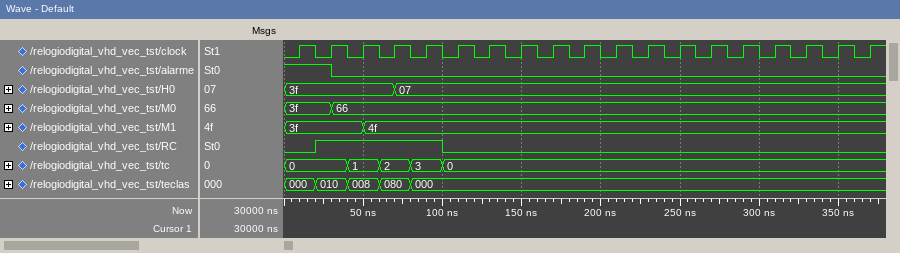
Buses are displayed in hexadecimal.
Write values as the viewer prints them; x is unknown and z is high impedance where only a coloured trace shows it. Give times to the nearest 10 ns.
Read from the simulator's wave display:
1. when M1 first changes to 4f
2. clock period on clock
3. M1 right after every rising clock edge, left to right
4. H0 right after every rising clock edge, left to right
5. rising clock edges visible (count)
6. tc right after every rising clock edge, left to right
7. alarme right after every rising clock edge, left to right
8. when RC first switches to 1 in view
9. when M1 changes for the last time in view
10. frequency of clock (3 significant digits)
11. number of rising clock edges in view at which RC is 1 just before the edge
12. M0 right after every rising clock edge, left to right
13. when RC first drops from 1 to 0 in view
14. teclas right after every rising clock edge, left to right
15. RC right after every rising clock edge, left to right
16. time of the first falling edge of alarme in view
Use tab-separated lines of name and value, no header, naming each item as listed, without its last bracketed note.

when M1 first changes to 4f	50 ns
clock period on clock	20 ns
M1 right after every rising clock edge, left to right	3f, 3f, 4f, 4f, 4f, 4f, 4f, 4f, 4f, 4f, 4f, 4f, 4f, 4f, 4f, 4f, 4f, 4f, 4f
H0 right after every rising clock edge, left to right	3f, 3f, 3f, 07, 07, 07, 07, 07, 07, 07, 07, 07, 07, 07, 07, 07, 07, 07, 07
rising clock edges visible	19
tc right after every rising clock edge, left to right	0, 0, 1, 2, 3, 0, 0, 0, 0, 0, 0, 0, 0, 0, 0, 0, 0, 0, 0
alarme right after every rising clock edge, left to right	1 0 0 0 0 0 0 0 0 0 0 0 0 0 0 0 0 0 0
when RC first switches to 1 in view	20 ns
when M1 changes for the last time in view	50 ns
frequency of clock	50.0 MHz
number of rising clock edges in view at which RC is 1 just before the edge	4
M0 right after every rising clock edge, left to right	3f, 66, 66, 66, 66, 66, 66, 66, 66, 66, 66, 66, 66, 66, 66, 66, 66, 66, 66
when RC first drops from 1 to 0 in view	100 ns
teclas right after every rising clock edge, left to right	000, 010, 008, 080, 000, 000, 000, 000, 000, 000, 000, 000, 000, 000, 000, 000, 000, 000, 000
RC right after every rising clock edge, left to right	0 1 1 1 1 0 0 0 0 0 0 0 0 0 0 0 0 0 0
time of the first falling edge of alarme in view	30 ns
